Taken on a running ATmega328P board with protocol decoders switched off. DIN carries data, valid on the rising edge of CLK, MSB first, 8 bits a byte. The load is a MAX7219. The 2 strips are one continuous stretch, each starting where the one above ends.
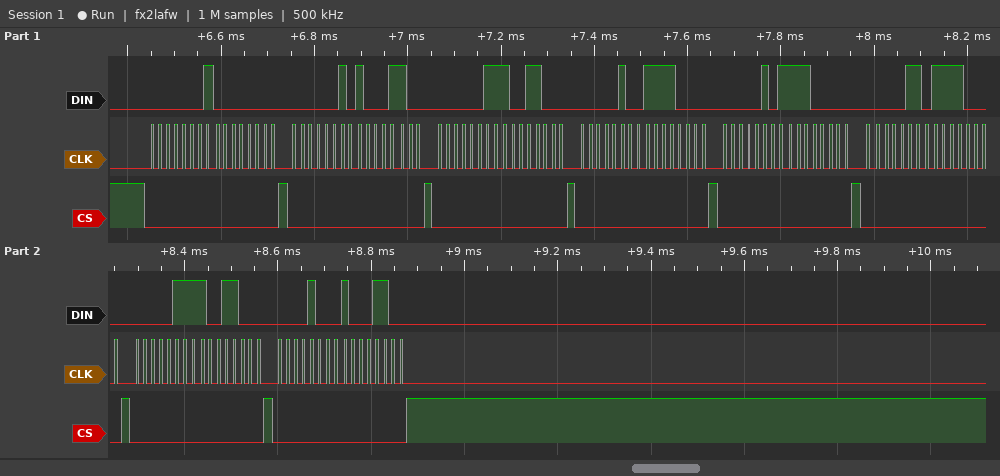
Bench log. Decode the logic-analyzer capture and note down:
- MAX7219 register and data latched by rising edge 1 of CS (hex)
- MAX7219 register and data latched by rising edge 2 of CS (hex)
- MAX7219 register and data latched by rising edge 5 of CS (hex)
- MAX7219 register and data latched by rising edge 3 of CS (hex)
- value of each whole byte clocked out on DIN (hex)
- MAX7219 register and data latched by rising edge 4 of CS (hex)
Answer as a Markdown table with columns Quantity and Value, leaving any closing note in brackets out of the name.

| Quantity | Value |
|---|---|
| MAX7219 register and data latched by rising edge 1 of CS | register 0x1, data 0x00 |
| MAX7219 register and data latched by rising edge 2 of CS | register 0x2, data 0x8C |
| MAX7219 register and data latched by rising edge 5 of CS | register 0x5, data 0xE0 |
| MAX7219 register and data latched by rising edge 3 of CS | register 0x3, data 0x98 |
| value of each whole byte clocked out on DIN | 0x01 0x00 0x02 0x8C 0x03 0x98 0x04 0xF0 0x05 0xE0 0x06 0xF0 0x07 0x98 0x08 0x8C |
| MAX7219 register and data latched by rising edge 4 of CS | register 0x4, data 0xF0 |
